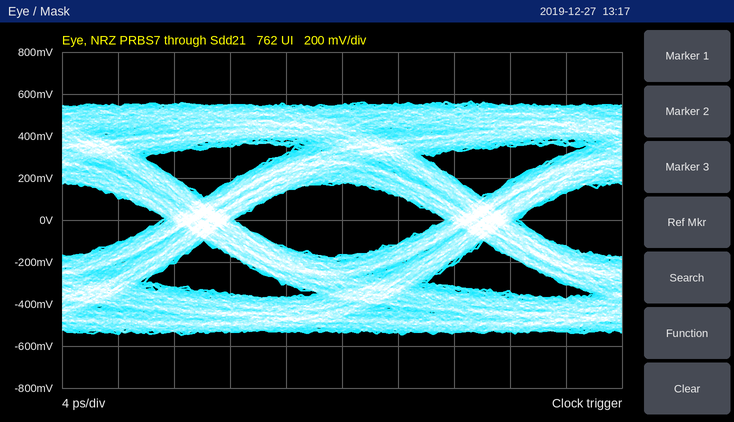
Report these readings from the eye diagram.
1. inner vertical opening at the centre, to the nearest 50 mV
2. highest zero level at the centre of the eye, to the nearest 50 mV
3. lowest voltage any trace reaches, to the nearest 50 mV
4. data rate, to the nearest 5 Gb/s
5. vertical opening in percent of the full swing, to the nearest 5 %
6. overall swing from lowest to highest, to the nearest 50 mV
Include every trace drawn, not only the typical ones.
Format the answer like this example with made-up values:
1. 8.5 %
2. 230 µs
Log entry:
1. 350 mV
2. -150 mV
3. -550 mV
4. 50 Gb/s
5. 30 %
6. 1.10 V
